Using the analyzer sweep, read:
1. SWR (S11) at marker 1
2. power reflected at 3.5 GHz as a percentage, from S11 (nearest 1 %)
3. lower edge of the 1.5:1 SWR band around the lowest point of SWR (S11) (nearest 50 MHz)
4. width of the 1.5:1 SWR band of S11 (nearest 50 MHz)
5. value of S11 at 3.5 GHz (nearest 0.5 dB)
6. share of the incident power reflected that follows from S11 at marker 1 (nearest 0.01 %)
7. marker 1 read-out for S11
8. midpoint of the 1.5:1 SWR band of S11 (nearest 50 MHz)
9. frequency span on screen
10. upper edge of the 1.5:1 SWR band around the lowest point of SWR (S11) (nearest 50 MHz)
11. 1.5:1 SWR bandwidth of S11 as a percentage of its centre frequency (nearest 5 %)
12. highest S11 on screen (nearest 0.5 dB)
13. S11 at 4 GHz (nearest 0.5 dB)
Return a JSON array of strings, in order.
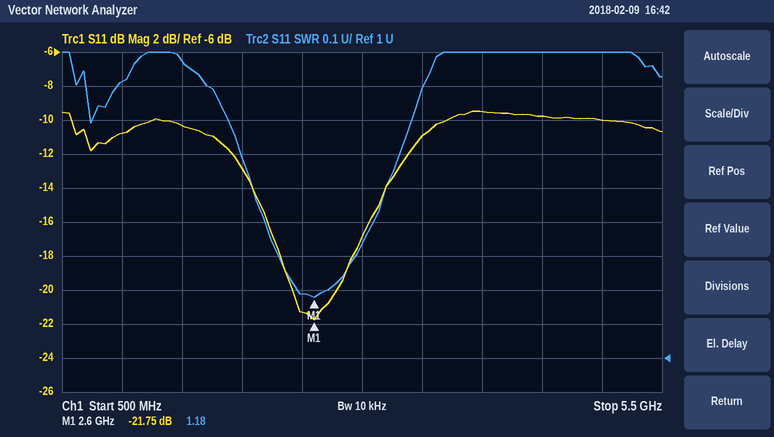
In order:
["1.18", "8 %", "2.10 GHz", "1.10 GHz", "-11.0 dB", "0.67 %", "-21.75 dB", "2.65 GHz", "5 GHz", "3.20 GHz", "40 %", "-9.5 dB", "-9.5 dB"]
